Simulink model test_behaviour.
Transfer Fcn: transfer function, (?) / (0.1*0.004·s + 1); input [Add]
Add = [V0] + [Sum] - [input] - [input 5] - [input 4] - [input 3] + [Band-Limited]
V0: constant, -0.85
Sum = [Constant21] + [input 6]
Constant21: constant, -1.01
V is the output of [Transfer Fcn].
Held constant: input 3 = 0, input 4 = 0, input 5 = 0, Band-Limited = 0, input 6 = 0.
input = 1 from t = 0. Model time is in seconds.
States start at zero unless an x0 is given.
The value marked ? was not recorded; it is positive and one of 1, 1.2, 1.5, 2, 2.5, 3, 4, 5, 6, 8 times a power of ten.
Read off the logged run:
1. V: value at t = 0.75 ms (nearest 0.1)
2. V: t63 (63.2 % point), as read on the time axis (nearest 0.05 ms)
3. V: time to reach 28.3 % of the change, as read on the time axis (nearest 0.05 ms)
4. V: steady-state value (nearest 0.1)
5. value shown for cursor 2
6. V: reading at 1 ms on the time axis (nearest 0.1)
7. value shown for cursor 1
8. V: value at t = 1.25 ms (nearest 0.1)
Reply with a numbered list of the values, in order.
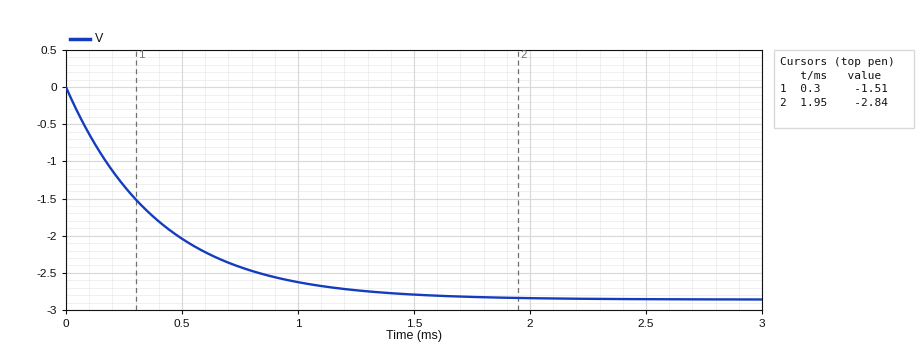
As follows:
1. -2.4
2. 0.40 ms
3. 0.15 ms
4. -2.9
5. -2.84
6. -2.6
7. -1.51
8. -2.7
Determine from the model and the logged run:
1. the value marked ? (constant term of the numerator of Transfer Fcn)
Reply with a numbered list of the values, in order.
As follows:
1. 1
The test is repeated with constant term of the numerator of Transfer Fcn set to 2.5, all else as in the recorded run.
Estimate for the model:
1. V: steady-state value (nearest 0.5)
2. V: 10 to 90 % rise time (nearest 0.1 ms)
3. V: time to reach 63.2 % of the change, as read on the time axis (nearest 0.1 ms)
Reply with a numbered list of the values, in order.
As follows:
1. -7.0
2. 0.9 ms
3. 0.4 ms
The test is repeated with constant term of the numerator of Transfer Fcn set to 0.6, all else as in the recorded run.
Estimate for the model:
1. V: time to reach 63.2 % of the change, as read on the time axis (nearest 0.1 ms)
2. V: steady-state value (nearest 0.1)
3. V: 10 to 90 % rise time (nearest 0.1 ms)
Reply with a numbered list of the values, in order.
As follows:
1. 0.4 ms
2. -1.7
3. 0.9 ms
